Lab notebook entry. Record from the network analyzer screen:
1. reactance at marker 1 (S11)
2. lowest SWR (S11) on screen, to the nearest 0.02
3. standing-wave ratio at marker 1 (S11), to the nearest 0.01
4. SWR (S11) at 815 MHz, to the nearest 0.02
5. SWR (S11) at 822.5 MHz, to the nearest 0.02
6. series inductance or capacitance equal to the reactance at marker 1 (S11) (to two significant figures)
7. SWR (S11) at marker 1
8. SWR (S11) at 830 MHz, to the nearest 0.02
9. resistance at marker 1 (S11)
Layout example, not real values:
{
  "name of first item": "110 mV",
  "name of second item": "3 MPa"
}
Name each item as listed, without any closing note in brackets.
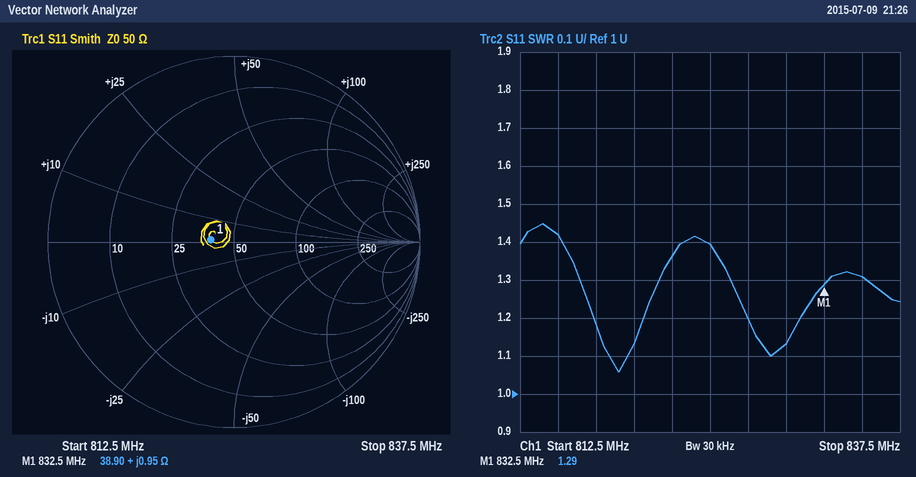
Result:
{
  "reactance at marker 1": "+0.95 Ω",
  "lowest SWR (S11) on screen, to the nearest 0.02": "1.06",
  "standing-wave ratio at marker 1 (S11), to the nearest 0.01": "1.29",
  "SWR (S11) at 815 MHz, to the nearest 0.02": "1.42",
  "SWR (S11) at 822.5 MHz, to the nearest 0.02": "1.36",
  "series inductance or capacitance equal to the reactance at marker 1 (S11)": "180 pH",
  "SWR (S11) at marker 1": "1.29",
  "SWR (S11) at 830 MHz, to the nearest 0.02": "1.14",
  "resistance at marker 1": "38.90 Ω"
}
